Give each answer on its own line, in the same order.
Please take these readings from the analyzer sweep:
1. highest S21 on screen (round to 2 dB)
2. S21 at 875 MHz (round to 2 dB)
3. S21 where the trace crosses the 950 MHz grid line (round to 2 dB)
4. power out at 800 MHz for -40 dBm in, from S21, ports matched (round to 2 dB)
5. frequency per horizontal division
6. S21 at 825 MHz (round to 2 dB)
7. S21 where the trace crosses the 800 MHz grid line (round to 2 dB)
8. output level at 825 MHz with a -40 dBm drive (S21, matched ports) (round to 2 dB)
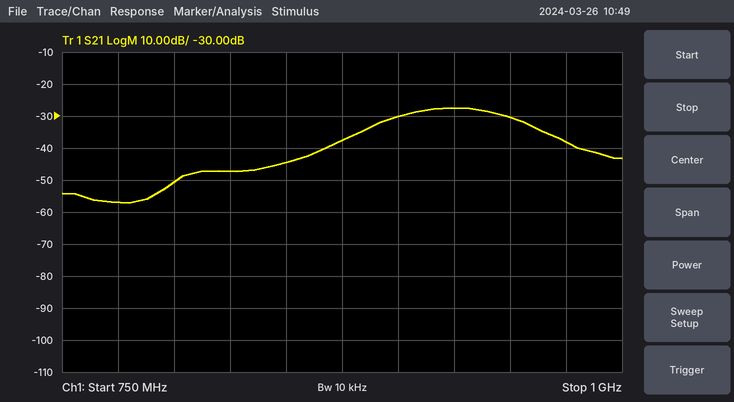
-28 dB
-38 dB
-30 dB
-90 dBm
25 MHz
-48 dB
-50 dB
-88 dBm
